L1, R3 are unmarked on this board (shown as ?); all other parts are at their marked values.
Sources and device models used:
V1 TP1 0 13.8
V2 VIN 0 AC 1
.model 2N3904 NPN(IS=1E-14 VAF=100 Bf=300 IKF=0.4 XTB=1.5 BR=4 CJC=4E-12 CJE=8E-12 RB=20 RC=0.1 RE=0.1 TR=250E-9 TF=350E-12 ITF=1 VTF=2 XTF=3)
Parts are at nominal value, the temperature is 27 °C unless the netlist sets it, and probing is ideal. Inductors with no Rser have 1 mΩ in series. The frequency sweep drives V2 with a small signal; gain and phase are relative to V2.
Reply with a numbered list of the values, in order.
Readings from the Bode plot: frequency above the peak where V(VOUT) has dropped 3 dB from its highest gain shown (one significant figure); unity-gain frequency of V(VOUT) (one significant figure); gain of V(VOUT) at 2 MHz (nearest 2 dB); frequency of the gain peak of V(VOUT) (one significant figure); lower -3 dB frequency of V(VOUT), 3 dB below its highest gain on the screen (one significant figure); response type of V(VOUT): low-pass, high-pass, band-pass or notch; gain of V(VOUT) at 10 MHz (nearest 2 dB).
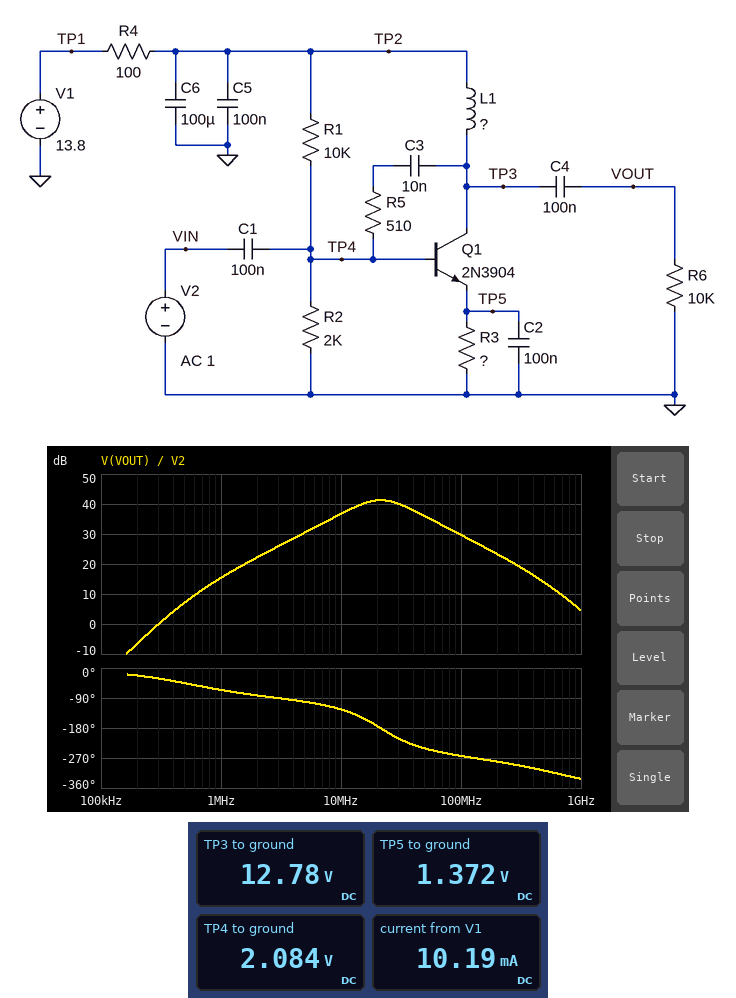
1. 40 MHz
2. 300 kHz
3. 22 dB
4. 20 MHz
5. 10 MHz
6. band-pass
7. 36 dB
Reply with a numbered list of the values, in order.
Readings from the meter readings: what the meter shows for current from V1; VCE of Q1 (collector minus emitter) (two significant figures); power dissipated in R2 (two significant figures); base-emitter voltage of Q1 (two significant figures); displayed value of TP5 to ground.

1. 10.19 mA
2. 11 V
3. 2.2 mW
4. 710 mV
5. 1.372 V
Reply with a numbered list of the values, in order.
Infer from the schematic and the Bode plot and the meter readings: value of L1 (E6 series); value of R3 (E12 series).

1. 3.3 µH
2. 150 Ω
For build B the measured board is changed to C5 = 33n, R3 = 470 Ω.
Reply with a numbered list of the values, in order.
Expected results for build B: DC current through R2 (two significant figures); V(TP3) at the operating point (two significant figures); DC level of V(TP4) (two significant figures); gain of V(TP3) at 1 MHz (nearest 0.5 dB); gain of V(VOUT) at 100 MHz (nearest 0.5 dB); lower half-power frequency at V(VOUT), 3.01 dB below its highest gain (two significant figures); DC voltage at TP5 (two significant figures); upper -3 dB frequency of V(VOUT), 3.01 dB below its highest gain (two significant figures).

1. 1.1 mA
2. 13 V
3. 2.2 V
4. 7.5 dB
5. 28.0 dB
6. 16 MHz
7. 1.5 V
8. 67 MHz
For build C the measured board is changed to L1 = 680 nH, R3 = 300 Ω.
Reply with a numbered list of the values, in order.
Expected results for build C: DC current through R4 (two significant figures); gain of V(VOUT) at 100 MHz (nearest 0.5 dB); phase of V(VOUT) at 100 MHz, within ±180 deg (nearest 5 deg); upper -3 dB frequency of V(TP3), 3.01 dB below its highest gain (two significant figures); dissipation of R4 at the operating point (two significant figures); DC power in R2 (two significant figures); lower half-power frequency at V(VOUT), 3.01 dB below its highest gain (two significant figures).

1. 6.0 mA
2. 30.0 dB
3. 125 deg
4. 100 MHz
5. 3.6 mW
6. 2.4 mW
7. 37 MHz
